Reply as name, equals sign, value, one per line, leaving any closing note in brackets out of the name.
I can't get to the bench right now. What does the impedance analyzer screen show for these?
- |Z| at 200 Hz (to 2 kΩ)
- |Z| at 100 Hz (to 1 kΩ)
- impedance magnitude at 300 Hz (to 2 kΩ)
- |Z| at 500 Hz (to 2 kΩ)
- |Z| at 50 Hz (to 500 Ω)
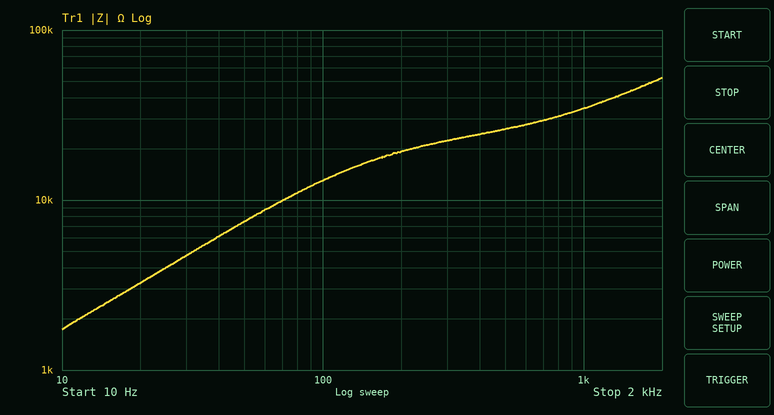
|Z| at 200 Hz = 20 kΩ
|Z| at 100 Hz = 13 kΩ
impedance magnitude at 300 Hz = 22 kΩ
|Z| at 500 Hz = 26 kΩ
|Z| at 50 Hz = 7.5 kΩ
